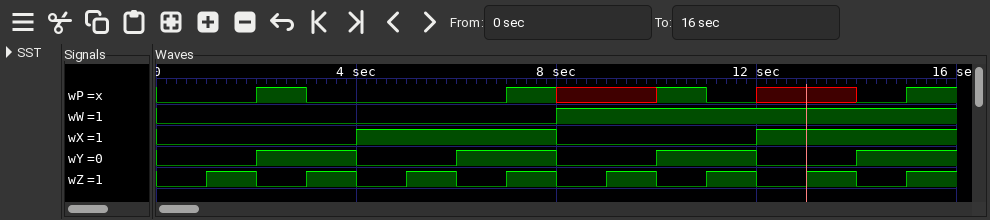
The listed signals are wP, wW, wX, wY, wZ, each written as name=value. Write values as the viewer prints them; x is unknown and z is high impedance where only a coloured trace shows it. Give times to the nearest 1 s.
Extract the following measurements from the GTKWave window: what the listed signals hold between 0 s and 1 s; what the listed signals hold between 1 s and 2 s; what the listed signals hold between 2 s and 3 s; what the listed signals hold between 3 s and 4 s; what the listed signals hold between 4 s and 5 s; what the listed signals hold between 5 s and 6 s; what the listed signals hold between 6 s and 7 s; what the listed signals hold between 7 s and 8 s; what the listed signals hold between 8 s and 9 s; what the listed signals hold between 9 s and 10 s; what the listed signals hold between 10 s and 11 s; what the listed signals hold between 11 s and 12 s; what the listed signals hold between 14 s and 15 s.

wP=0, wW=0, wX=0, wY=0, wZ=0
wP=0, wW=0, wX=0, wY=0, wZ=1
wP=1, wW=0, wX=0, wY=1, wZ=0
wP=0, wW=0, wX=0, wY=1, wZ=1
wP=0, wW=0, wX=1, wY=0, wZ=0
wP=0, wW=0, wX=1, wY=0, wZ=1
wP=0, wW=0, wX=1, wY=1, wZ=0
wP=1, wW=0, wX=1, wY=1, wZ=1
wP=x, wW=1, wX=0, wY=0, wZ=0
wP=x, wW=1, wX=0, wY=0, wZ=1
wP=1, wW=1, wX=0, wY=1, wZ=0
wP=0, wW=1, wX=0, wY=1, wZ=1
wP=0, wW=1, wX=1, wY=1, wZ=0
